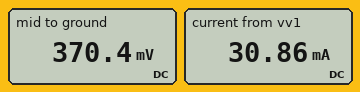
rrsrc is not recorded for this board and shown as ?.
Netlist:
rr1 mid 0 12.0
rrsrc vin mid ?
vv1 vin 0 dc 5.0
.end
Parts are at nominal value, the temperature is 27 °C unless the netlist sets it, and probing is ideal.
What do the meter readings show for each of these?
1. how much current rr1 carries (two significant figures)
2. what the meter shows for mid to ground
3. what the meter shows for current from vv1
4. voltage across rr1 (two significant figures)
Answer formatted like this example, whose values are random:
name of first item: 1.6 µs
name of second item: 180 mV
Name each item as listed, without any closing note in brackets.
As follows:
how much current rr1 carries: 31 mA
what the meter shows for mid to ground: 370.4 mV
what the meter shows for current from vv1: 30.86 mA
voltage across rr1: 370 mV
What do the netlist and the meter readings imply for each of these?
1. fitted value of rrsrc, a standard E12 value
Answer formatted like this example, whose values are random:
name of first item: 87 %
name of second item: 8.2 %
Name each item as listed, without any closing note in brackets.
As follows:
fitted value of rrsrc, a standard E12 value: 150 Ω
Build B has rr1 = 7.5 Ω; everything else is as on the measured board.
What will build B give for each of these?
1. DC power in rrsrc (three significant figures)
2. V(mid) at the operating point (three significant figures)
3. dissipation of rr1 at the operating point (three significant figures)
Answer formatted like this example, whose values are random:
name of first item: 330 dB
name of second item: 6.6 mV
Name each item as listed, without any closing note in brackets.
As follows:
DC power in rrsrc: 151 mW
V(mid) at the operating point: 238 mV
dissipation of rr1 at the operating point: 7.56 mW
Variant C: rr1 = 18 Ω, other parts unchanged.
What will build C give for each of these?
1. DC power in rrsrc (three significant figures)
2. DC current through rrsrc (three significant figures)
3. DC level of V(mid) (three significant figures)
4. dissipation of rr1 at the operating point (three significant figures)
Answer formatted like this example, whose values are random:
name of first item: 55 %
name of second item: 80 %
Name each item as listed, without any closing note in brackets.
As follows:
DC power in rrsrc: 133 mW
DC current through rrsrc: 29.8 mA
DC level of V(mid): 536 mV
dissipation of rr1 at the operating point: 15.9 mW
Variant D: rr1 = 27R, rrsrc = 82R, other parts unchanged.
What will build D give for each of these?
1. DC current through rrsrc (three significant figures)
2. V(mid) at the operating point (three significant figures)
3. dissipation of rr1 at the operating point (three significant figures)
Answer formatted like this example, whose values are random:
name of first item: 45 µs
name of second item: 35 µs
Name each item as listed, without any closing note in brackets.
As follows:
DC current through rrsrc: 45.9 mA
V(mid) at the operating point: 1.24 V
dissipation of rr1 at the operating point: 56.8 mW
